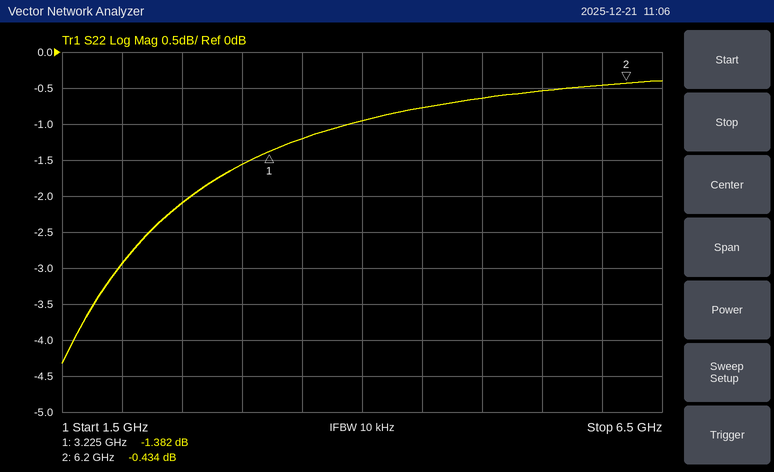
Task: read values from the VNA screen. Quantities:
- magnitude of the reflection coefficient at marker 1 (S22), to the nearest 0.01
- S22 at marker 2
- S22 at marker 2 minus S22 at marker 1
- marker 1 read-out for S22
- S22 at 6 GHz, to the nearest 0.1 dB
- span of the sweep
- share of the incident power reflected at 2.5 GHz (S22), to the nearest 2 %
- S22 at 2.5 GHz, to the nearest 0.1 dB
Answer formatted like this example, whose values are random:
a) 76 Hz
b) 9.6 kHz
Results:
a) 0.85
b) -0.434 dB
c) 0.948 dB
d) -1.382 dB
e) -0.5 dB
f) 5 GHz
g) 62 %
h) -2.1 dB
